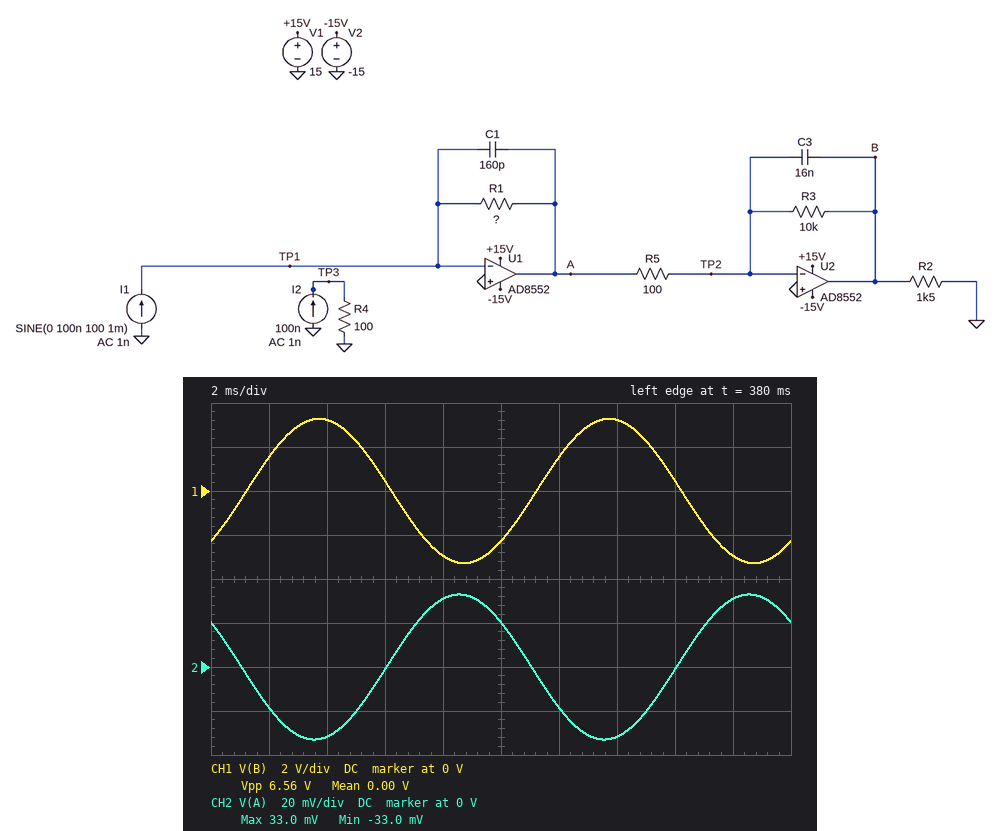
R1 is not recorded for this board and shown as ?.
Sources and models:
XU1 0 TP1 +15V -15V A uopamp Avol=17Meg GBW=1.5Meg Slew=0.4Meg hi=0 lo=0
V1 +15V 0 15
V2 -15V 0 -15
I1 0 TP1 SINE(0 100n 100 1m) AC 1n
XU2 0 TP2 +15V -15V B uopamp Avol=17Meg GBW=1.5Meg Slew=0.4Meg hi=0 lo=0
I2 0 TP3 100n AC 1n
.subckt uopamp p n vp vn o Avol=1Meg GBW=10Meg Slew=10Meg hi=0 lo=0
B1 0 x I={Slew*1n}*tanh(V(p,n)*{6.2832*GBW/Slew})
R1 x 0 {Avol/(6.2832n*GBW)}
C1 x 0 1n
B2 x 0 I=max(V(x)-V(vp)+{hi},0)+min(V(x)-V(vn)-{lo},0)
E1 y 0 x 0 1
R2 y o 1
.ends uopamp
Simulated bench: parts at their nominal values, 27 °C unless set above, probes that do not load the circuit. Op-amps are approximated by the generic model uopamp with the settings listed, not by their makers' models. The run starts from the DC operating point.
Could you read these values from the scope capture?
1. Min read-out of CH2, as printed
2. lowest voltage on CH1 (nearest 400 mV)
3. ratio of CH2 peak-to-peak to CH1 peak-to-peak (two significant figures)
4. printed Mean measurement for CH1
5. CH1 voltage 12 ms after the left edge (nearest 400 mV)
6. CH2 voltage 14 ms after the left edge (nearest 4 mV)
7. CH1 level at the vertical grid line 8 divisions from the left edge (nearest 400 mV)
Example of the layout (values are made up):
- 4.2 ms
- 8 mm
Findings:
- -33.0 mV
- -3.2 V
- 0.010
- 0.00 V
- 1.6 V
- -32 mV
- 400 mV
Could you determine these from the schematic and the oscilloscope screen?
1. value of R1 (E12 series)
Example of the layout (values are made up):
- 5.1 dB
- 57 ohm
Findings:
- 330 kΩ
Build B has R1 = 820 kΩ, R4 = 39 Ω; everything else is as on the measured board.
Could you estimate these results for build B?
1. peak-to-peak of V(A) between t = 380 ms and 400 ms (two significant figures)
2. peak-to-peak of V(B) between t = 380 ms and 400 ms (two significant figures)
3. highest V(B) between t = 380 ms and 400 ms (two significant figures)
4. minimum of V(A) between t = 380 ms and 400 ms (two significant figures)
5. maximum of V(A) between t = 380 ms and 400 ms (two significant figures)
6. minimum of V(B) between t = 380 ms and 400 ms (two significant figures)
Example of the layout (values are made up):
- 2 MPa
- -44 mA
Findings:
- 160 mV
- 16 V
- 8.1 V
- -82 mV
- 82 mV
- -8.1 V
